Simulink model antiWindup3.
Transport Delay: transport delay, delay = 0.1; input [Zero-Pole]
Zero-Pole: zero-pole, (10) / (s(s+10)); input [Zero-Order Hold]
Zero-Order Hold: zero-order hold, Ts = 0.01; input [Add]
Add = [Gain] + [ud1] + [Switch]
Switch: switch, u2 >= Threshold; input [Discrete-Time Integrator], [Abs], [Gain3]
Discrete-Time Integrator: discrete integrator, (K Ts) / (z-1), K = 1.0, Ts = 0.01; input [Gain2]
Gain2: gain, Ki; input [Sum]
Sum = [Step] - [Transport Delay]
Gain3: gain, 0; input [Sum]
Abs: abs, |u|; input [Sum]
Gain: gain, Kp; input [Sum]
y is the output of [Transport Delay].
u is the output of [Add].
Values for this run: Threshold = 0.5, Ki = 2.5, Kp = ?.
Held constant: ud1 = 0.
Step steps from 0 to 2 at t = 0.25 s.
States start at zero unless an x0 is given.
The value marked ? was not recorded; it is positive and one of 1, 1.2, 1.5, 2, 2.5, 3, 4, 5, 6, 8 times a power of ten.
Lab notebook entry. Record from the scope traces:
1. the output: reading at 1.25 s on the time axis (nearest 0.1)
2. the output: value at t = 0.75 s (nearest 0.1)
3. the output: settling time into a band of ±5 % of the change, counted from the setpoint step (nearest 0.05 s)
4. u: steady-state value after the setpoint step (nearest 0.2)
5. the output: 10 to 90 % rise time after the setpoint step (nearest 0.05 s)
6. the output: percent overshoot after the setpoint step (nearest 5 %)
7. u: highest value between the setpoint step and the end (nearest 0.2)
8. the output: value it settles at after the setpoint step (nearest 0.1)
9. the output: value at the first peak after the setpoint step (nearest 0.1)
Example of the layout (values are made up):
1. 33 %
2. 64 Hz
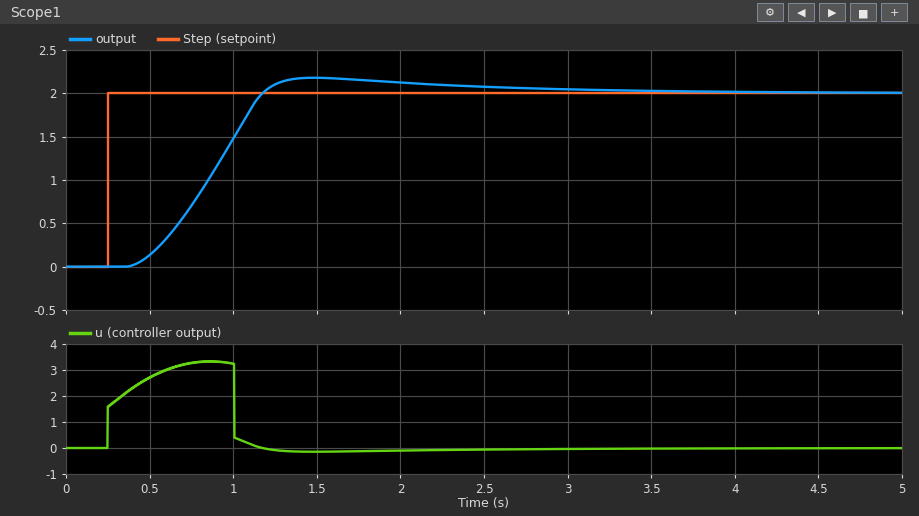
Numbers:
1. 2.1
2. 0.7
3. 1.95 s
4. 0.0
5. 0.55 s
6. 10 %
7. 3.4
8. 2.0
9. 2.2
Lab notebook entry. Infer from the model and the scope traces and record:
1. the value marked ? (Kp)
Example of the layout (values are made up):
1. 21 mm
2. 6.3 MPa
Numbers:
1. 0.8
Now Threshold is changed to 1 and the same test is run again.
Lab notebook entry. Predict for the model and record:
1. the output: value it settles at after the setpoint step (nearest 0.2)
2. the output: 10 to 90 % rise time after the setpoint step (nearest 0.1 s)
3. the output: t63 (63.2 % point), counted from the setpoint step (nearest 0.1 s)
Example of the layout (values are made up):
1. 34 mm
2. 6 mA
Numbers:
1. 2.0
2. 0.8 s
3. 0.7 s
